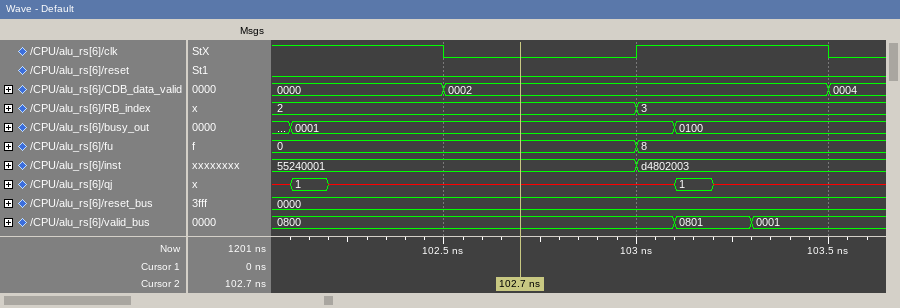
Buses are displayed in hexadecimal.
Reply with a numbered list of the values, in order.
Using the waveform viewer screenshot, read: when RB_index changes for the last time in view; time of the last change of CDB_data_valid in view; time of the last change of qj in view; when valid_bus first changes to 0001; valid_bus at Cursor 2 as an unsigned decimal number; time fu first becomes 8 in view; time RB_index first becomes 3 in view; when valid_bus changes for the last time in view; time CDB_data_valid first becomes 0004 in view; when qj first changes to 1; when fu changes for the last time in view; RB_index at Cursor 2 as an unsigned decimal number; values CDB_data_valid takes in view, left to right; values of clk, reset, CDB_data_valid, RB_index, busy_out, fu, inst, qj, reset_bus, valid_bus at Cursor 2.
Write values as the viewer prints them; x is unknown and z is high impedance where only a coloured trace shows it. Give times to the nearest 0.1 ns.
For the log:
1. 103 ns
2. 103.5 ns
3. 103.2 ns
4. 103.3 ns
5. 2048
6. 103 ns
7. 103 ns
8. 103.3 ns
9. 103.5 ns
10. 102.1 ns
11. 103 ns
12. 2
13. 0000, 0002, 0004
14. clk=0, reset=0, CDB_data_valid=0002, RB_index=2, busy_out=0001, fu=0, inst=55240001, qj=x, reset_bus=0000, valid_bus=0800
